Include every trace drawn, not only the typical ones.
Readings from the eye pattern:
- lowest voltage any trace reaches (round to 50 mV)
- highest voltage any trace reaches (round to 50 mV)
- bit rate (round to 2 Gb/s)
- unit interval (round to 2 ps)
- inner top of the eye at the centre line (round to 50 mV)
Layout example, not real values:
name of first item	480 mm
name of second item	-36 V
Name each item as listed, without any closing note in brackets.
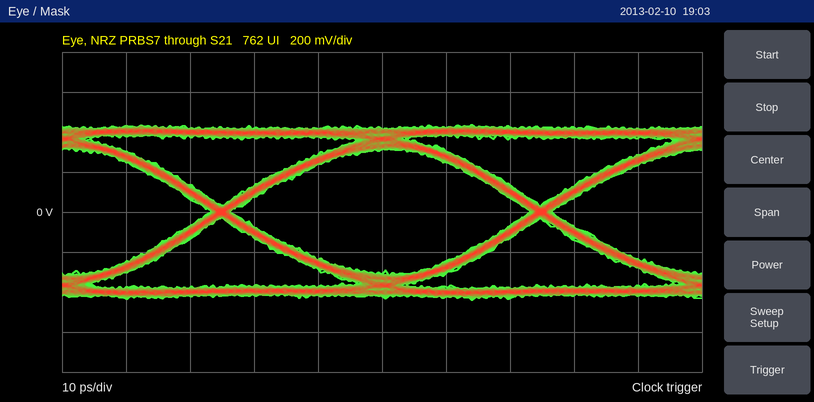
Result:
lowest voltage any trace reaches	-450 mV
highest voltage any trace reaches	450 mV
bit rate	20 Gb/s
unit interval	50 ps
inner top of the eye at the centre line	300 mV
